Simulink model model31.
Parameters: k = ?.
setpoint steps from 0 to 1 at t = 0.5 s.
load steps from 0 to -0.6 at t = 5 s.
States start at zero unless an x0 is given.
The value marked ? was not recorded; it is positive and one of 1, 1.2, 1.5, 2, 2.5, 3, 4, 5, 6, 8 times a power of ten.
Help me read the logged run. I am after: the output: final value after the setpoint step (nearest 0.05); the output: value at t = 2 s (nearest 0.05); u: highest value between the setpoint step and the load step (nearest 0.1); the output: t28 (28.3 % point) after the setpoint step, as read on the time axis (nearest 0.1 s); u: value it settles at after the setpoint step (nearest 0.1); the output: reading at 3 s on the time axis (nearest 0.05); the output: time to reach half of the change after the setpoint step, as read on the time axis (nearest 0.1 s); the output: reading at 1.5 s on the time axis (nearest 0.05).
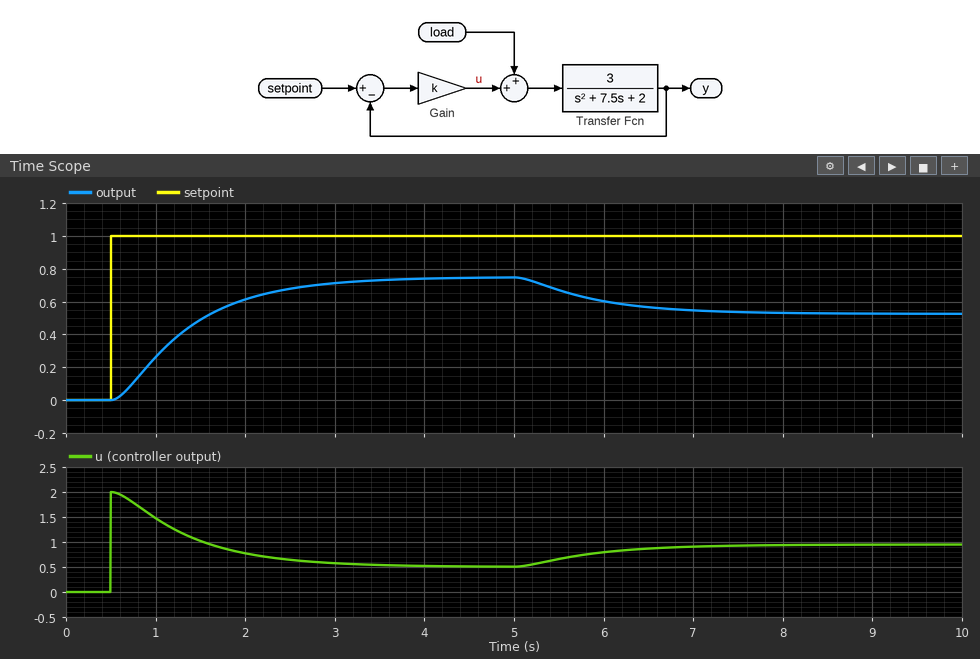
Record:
0.75
0.60
2.0
0.9 s
0.5
0.70
1.2 s
0.50
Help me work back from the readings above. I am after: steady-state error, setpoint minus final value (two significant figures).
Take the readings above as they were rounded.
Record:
0.25
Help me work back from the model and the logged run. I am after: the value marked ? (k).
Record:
2
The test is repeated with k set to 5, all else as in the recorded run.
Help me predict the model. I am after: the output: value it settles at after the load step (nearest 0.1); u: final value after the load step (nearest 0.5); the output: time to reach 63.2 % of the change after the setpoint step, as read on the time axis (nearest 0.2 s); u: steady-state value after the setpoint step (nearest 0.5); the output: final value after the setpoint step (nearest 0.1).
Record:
0.8
1.0
1.0 s
0.5
0.9
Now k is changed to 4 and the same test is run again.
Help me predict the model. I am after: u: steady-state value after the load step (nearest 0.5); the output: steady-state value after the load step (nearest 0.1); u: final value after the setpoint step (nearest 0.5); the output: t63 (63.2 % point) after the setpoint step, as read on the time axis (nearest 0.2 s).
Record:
1.0
0.7
0.5
1.0 s
